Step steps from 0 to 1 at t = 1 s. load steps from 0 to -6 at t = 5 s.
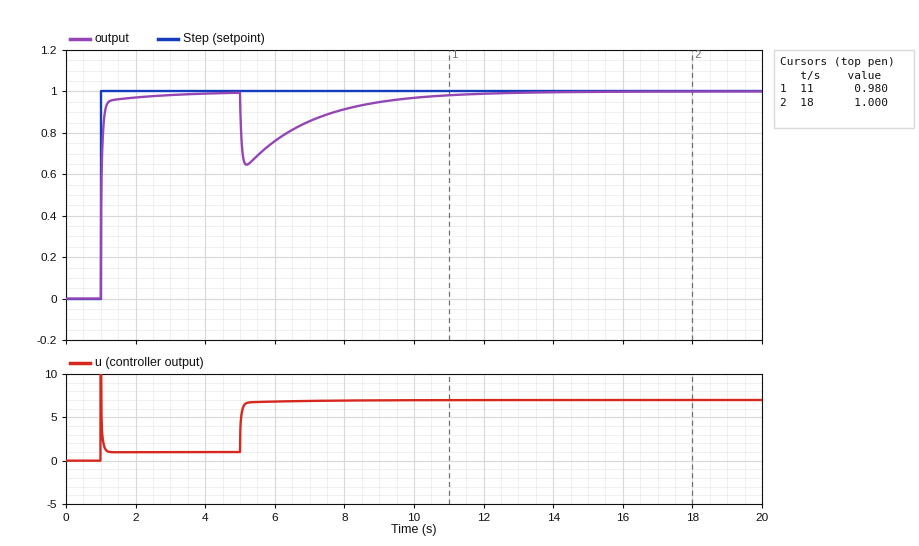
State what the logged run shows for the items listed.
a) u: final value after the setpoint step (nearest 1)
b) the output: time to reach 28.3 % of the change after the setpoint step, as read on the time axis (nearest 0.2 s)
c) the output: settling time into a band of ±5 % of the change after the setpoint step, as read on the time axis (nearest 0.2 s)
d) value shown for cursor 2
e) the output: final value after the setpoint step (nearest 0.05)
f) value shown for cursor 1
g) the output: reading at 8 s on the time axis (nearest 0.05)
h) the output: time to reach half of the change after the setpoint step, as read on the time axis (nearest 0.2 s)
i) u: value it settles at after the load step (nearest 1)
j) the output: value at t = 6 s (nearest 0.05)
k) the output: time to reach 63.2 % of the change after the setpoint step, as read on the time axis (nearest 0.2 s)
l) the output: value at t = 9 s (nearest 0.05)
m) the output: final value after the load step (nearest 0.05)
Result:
1
1.0 s
1.2 s
1.000
1.00
0.980
0.90
1.0 s
7
0.75
1.0 s
0.95
1.00
